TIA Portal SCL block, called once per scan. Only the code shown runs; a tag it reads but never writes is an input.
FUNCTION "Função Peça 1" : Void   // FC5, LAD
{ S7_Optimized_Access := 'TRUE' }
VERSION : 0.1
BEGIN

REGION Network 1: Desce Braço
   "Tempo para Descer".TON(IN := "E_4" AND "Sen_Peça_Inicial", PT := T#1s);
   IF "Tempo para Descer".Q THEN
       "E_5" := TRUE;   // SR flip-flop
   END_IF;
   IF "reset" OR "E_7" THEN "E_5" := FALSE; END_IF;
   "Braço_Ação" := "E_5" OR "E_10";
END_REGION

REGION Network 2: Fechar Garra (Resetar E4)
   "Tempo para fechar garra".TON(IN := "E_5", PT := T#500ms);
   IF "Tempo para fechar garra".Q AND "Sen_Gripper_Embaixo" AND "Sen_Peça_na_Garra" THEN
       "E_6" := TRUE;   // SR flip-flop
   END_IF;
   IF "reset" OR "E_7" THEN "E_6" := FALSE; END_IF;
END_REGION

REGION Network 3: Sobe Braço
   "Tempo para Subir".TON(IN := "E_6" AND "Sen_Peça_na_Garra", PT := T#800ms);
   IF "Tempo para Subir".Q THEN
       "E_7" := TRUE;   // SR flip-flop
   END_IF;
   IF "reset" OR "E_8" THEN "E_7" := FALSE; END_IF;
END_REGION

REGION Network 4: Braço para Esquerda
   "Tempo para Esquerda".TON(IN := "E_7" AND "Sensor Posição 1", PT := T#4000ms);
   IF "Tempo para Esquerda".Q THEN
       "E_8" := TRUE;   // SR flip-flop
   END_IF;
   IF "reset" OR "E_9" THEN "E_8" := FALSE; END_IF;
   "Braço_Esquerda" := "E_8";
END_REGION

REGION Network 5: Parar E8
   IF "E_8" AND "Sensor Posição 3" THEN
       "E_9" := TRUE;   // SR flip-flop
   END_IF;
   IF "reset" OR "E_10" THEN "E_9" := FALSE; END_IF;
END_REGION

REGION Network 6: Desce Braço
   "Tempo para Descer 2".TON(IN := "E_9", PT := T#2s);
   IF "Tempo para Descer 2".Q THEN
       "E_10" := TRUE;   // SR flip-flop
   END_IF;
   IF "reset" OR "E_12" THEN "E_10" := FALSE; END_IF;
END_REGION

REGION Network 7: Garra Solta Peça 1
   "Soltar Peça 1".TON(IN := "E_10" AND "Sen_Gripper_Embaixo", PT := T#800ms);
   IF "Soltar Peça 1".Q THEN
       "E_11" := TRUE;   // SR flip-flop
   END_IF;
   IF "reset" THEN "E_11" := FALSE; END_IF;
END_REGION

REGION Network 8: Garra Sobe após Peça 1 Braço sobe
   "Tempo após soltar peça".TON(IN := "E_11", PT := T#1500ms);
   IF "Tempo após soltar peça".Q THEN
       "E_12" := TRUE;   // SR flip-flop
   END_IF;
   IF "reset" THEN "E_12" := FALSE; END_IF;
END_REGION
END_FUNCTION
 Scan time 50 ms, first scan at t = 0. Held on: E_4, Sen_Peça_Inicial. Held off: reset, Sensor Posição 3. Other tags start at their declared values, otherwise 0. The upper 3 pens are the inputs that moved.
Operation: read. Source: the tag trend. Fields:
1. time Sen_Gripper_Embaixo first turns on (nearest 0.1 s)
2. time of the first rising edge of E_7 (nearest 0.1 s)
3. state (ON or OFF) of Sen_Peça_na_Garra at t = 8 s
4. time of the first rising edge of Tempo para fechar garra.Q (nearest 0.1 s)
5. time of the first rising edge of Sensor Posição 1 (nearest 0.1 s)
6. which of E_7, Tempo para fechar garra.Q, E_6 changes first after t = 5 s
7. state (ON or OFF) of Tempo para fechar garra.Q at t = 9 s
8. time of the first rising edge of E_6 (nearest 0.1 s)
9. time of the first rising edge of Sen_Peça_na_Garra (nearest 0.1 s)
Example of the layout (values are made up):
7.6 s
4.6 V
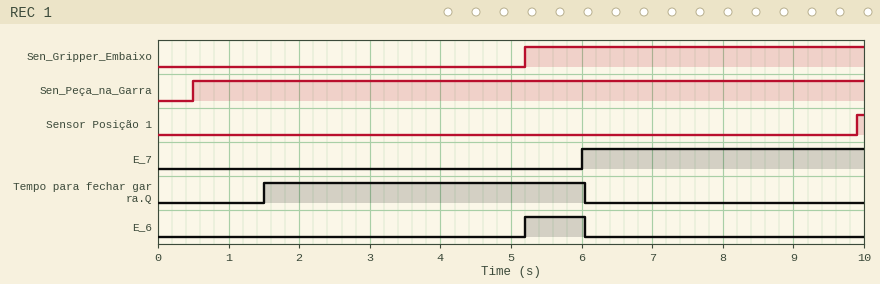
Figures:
5.2 s
6.0 s
ON
1.5 s
9.9 s
E_6
OFF
5.2 s
0.5 s
